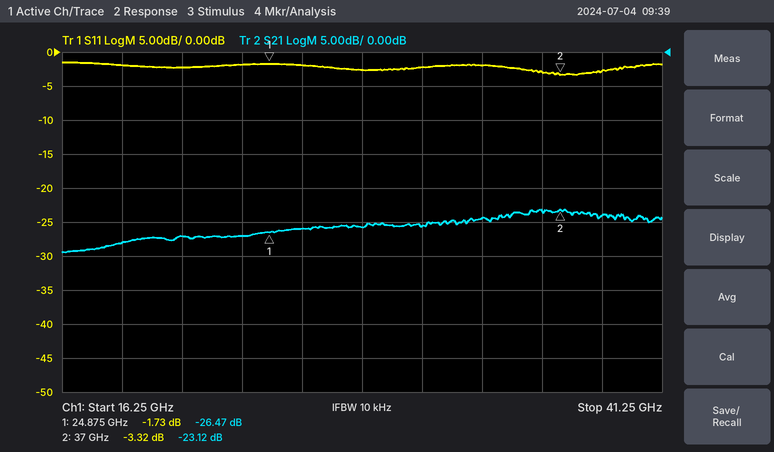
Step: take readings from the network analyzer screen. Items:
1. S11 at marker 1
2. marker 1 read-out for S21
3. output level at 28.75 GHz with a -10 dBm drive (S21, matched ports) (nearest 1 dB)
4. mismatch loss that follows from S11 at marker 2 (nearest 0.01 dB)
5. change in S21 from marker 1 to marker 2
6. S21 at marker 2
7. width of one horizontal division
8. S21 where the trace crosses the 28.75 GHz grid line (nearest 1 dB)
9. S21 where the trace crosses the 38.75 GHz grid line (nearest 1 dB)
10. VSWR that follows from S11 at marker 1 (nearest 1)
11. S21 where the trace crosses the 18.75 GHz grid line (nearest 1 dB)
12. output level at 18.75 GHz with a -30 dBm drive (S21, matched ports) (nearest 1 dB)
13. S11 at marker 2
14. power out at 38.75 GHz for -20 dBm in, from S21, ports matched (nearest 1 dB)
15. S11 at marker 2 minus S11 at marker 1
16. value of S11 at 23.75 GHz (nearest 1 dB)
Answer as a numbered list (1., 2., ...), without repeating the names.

1. -1.73 dB
2. -26.47 dB
3. -36 dBm
4. 2.72 dB
5. 3.35 dB
6. -23.12 dB
7. 2.5 GHz
8. -26 dB
9. -24 dB
10. 10
11. -28 dB
12. -58 dBm
13. -3.32 dB
14. -44 dBm
15. -1.59 dB
16. -2 dB
